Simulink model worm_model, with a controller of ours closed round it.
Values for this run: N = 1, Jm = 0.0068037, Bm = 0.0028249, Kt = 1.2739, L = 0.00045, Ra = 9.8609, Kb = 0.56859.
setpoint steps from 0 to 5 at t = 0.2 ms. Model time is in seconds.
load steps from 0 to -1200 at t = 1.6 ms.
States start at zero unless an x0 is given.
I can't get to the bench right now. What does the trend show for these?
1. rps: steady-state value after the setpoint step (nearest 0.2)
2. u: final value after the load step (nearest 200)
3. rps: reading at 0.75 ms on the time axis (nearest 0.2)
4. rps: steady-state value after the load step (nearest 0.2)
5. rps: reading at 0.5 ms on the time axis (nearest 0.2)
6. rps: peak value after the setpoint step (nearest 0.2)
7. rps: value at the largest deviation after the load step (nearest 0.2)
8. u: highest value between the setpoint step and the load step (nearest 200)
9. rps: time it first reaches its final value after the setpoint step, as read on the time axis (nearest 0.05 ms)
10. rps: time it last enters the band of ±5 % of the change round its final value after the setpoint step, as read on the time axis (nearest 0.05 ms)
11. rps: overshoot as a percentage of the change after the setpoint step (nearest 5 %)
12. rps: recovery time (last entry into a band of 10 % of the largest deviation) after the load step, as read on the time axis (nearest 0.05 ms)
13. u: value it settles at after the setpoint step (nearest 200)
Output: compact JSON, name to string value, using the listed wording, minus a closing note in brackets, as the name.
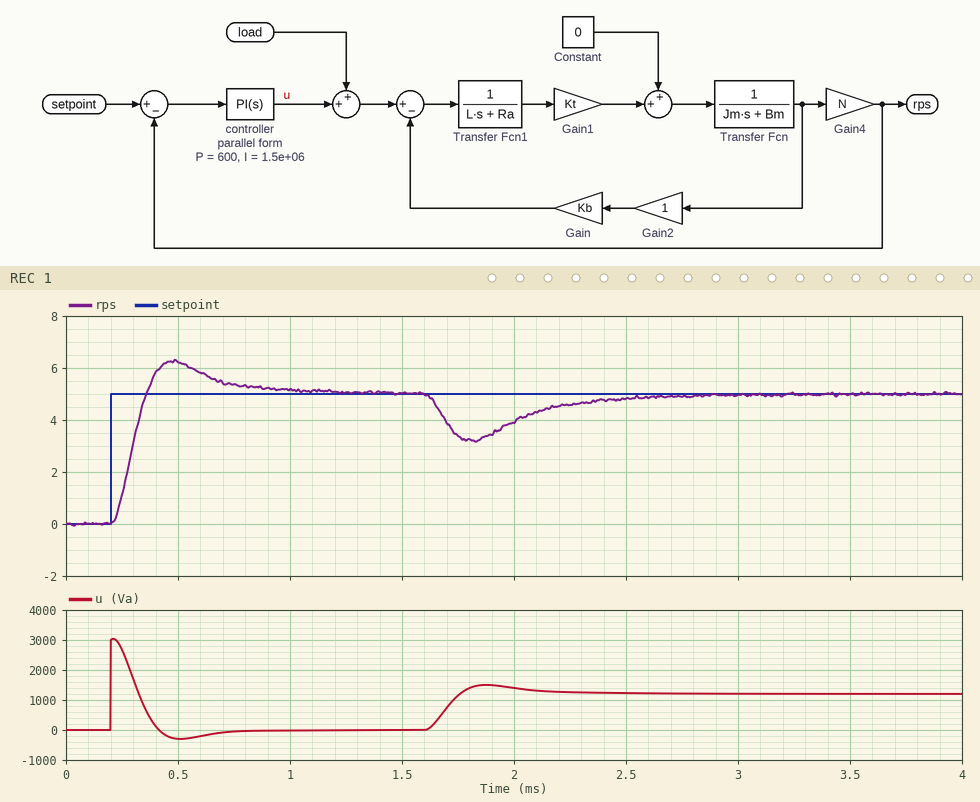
{"rps: steady-state value after the setpoint step": "5.0", "u: final value after the load step": "1200", "rps: reading at 0.75 ms on the time axis": "5.4", "rps: steady-state value after the load step": "5.0", "rps: reading at 0.5 ms on the time axis": "6.2", "rps: peak value after the setpoint step": "6.2", "rps: value at the largest deviation after the load step": "3.2", "u: highest value between the setpoint step and the load step": "3000", "rps: time it first reaches its final value after the setpoint step, as read on the time axis": "0.35 ms", "rps: time it last enters the band of ±5 % of the change round its final value after the setpoint step, as read on the time axis": "0.85 ms", "rps: overshoot as a percentage of the change after the setpoint step": "25 %", "rps: recovery time (last entry into a band of 10 % of the largest deviation) after the load step, as read on the time axis": "2.50 ms", "u: value it settles at after the setpoint step": "0"}
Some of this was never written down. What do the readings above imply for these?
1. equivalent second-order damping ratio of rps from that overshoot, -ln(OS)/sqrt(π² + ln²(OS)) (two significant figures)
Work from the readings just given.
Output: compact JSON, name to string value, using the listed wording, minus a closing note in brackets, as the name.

{"equivalent second-order damping ratio of rps from that overshoot, -ln(OS)/sqrt(π² + ln²(OS))": "0.40"}
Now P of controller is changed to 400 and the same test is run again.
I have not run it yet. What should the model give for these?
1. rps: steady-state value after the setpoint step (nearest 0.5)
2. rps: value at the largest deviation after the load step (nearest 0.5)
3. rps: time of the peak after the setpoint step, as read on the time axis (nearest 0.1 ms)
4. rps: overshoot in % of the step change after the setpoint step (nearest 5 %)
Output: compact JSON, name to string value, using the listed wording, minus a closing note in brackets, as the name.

{"rps: steady-state value after the setpoint step": "5.0", "rps: value at the largest deviation after the load step": "2.5", "rps: time of the peak after the setpoint step, as read on the time axis": "0.6 ms", "rps: overshoot in % of the step change after the setpoint step": "35 %"}
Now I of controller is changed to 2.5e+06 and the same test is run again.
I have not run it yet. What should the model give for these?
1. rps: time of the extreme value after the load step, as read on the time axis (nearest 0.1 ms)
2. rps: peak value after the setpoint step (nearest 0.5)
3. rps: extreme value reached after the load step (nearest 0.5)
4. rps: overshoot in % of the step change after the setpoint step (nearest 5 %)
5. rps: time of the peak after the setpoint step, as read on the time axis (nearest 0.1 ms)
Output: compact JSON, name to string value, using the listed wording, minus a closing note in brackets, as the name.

{"rps: time of the extreme value after the load step, as read on the time axis": "1.8 ms", "rps: peak value after the setpoint step": "7.0", "rps: extreme value reached after the load step": "3.5", "rps: overshoot in % of the step change after the setpoint step": "35 %", "rps: time of the peak after the setpoint step, as read on the time axis": "0.5 ms"}
